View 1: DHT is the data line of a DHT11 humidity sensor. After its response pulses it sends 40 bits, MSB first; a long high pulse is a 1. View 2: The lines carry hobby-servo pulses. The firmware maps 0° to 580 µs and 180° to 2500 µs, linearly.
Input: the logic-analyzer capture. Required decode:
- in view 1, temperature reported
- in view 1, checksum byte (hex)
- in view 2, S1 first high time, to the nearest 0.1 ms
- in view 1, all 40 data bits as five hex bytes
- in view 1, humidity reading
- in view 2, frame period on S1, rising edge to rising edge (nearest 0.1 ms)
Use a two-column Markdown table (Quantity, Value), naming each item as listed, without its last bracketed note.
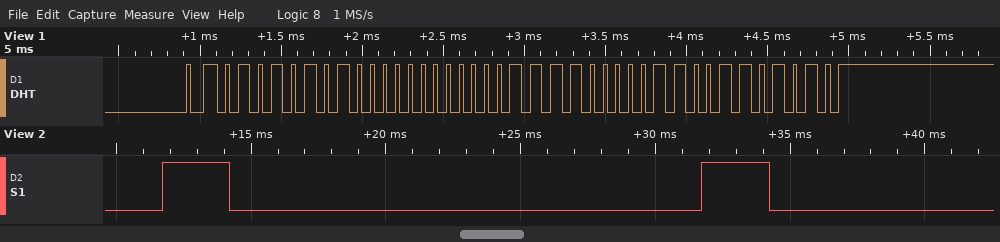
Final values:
| Quantity | Value |
|---|---|
| in view 1, temperature reported | 15.6 °C |
| in view 1, checksum byte | 0x6A |
| in view 2, S1 first high time, to the nearest 0.1 ms | 2.5 ms |
| in view 1, all 40 data bits as five hex bytes | 55 00 0F 06 6A |
| in view 1, humidity reading | 85 % |
| in view 2, frame period on S1, rising edge to rising edge | 20.0 ms |
